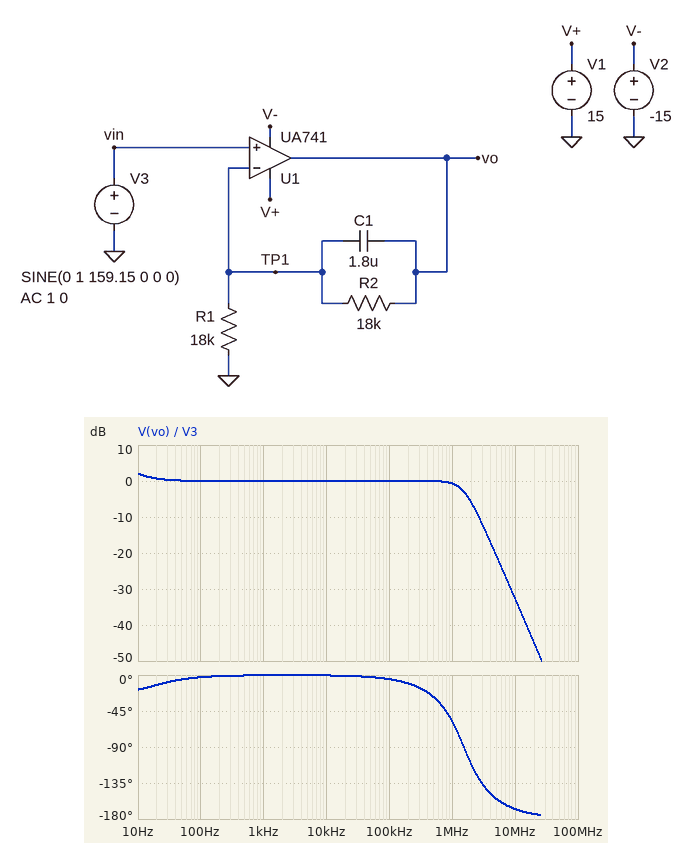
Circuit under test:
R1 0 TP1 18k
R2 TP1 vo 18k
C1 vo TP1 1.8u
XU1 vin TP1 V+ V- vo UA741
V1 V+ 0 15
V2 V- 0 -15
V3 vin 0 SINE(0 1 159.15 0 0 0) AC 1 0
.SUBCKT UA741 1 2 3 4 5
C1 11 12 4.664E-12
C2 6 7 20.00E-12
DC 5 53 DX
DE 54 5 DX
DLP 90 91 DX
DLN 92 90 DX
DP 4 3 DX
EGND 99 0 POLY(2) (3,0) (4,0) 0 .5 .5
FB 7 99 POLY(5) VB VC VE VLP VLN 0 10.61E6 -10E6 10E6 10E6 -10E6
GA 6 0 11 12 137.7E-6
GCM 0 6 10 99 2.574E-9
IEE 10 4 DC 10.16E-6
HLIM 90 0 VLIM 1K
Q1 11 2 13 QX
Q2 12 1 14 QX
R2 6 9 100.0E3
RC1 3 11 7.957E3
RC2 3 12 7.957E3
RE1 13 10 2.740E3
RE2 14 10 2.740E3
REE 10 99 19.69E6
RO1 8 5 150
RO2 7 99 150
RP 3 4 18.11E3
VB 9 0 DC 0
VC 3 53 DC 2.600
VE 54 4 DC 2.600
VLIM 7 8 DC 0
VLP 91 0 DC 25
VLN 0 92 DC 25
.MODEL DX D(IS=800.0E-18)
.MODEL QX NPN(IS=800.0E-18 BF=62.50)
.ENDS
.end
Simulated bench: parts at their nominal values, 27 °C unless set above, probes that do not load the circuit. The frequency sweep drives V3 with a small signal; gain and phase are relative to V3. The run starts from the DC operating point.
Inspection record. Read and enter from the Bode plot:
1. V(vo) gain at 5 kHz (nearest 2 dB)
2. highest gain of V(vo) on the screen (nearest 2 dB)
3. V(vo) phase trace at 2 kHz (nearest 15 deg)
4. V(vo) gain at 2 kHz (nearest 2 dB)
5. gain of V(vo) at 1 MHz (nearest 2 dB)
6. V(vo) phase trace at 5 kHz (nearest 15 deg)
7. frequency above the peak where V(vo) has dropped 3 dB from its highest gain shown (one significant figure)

0 dB
2 dB
0 deg
0 dB
0 dB
0 deg
1 MHz
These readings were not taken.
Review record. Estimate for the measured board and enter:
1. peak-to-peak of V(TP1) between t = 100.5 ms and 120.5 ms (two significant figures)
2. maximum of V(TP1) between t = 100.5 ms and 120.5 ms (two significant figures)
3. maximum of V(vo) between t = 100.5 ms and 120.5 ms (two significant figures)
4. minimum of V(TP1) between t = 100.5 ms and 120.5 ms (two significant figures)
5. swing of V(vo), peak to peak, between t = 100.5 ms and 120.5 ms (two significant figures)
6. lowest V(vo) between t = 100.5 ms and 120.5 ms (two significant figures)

2.0 V
1.0 V
1.0 V
-1.0 V
2.0 V
-1.0 V
